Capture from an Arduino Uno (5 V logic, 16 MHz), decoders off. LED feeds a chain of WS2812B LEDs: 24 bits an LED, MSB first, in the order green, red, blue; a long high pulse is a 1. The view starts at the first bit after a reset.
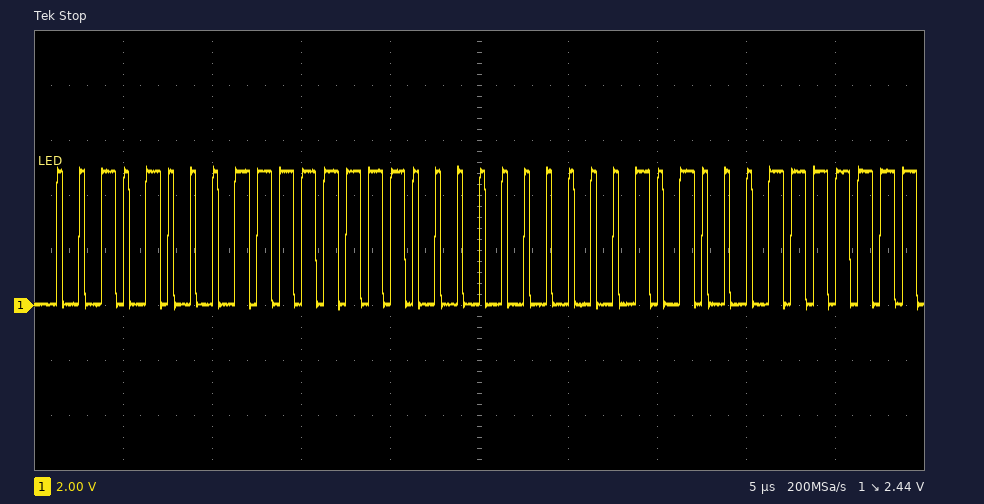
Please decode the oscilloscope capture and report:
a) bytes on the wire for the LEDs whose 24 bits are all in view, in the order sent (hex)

28 FF 00
